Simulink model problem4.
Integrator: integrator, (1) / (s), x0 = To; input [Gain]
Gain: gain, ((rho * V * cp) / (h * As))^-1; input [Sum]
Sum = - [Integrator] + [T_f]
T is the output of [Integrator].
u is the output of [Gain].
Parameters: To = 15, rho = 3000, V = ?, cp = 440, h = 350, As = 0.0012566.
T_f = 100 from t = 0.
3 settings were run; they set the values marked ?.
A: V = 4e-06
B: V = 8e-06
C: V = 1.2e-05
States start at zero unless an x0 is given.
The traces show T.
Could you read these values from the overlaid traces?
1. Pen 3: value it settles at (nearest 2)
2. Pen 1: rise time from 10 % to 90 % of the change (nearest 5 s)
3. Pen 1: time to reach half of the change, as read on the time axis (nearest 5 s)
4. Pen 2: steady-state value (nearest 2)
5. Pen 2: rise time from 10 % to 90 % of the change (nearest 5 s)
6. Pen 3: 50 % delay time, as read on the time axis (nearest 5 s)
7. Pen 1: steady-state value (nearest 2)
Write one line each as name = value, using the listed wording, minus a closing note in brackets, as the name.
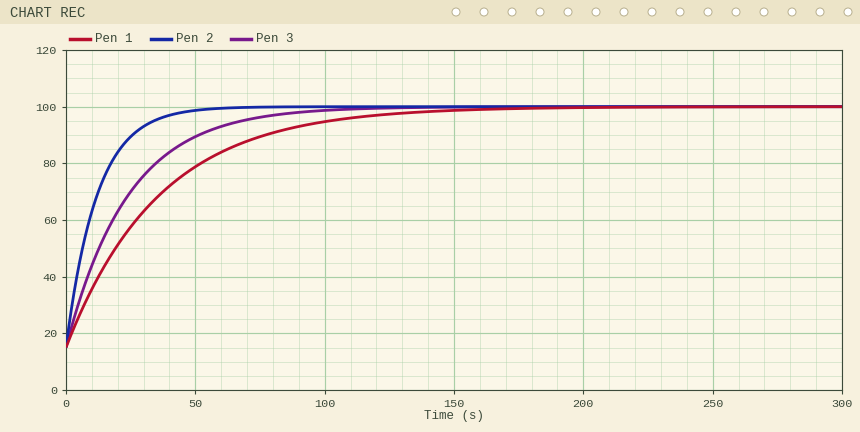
Pen 3: value it settles at = 100
Pen 1: rise time from 10 % to 90 % of the change = 80 s
Pen 1: time to reach half of the change, as read on the time axis = 25 s
Pen 2: steady-state value = 100
Pen 2: rise time from 10 % to 90 % of the change = 25 s
Pen 3: 50 % delay time, as read on the time axis = 15 s
Pen 1: steady-state value = 100
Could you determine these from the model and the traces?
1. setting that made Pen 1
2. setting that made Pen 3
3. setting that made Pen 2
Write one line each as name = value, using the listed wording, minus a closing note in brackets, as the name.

setting that made Pen 1 = C
setting that made Pen 3 = B
setting that made Pen 2 = A
